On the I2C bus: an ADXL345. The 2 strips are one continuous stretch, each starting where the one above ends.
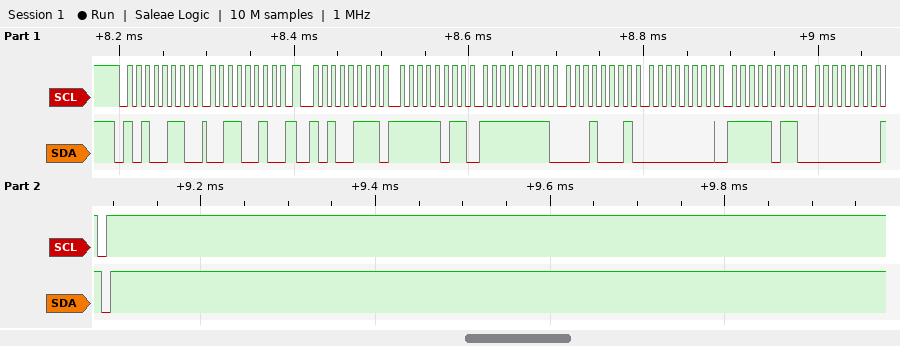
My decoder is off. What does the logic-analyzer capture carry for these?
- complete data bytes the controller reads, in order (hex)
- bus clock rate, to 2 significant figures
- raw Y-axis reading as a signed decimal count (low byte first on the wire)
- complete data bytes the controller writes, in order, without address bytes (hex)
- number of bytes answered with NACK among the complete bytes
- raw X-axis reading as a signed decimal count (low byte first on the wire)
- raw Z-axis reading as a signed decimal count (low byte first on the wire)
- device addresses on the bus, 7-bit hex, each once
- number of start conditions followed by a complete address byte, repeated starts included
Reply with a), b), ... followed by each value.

a) FB FF 11 00 FB 00
b) 100 kHz
c) 17
d) 32
e) 1
f) -5
g) 251
h) 0x53
i) 2
